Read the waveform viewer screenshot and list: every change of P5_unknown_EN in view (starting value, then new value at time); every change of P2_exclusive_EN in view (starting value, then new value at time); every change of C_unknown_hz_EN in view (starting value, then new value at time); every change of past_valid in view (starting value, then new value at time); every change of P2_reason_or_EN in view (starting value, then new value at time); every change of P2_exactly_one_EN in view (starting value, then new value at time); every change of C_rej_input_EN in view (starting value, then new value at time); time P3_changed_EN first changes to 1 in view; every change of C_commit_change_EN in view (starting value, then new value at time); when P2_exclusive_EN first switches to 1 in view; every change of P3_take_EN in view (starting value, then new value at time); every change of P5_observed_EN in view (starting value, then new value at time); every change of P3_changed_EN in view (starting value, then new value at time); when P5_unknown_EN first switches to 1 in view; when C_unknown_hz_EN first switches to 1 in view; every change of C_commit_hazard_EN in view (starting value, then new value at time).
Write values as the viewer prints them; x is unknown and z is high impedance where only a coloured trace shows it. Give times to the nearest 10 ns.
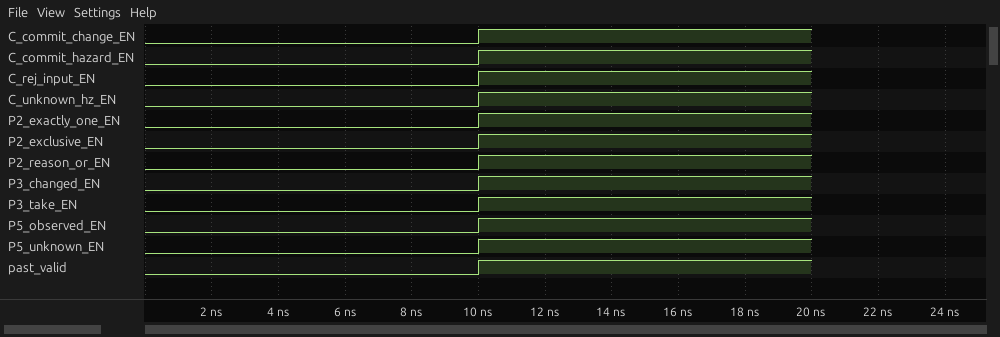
0, 1 at 10 ns
0, 1 at 10 ns
0, 1 at 10 ns
0, 1 at 10 ns
0, 1 at 10 ns
0, 1 at 10 ns
0, 1 at 10 ns
10 ns
0, 1 at 10 ns
10 ns
0, 1 at 10 ns
0, 1 at 10 ns
0, 1 at 10 ns
10 ns
10 ns
0, 1 at 10 ns
